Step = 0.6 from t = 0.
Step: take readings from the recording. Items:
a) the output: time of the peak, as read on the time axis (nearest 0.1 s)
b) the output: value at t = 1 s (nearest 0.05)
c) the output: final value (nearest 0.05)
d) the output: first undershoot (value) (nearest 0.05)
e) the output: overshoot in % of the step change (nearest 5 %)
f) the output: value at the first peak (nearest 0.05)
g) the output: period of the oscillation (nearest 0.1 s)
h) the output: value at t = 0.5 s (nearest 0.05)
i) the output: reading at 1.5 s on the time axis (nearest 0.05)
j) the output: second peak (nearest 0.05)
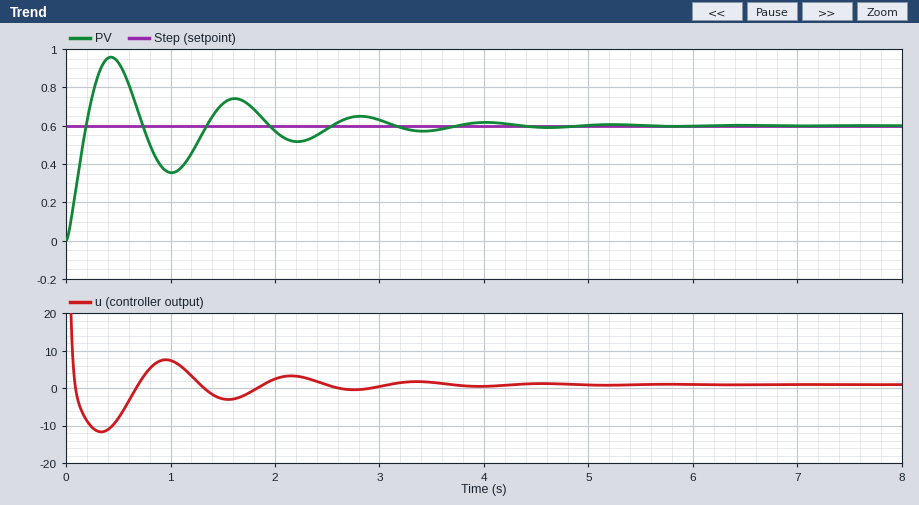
0.4 s
0.35
0.60
0.35
60 %
0.95
1.2 s
0.95
0.70
0.75
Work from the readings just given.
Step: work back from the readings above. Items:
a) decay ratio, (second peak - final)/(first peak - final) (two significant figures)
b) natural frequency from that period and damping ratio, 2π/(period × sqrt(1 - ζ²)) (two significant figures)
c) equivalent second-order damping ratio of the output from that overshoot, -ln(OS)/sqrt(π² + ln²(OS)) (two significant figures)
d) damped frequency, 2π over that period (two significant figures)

0.43
5.3 rad/s
0.16
5.2 rad/s
